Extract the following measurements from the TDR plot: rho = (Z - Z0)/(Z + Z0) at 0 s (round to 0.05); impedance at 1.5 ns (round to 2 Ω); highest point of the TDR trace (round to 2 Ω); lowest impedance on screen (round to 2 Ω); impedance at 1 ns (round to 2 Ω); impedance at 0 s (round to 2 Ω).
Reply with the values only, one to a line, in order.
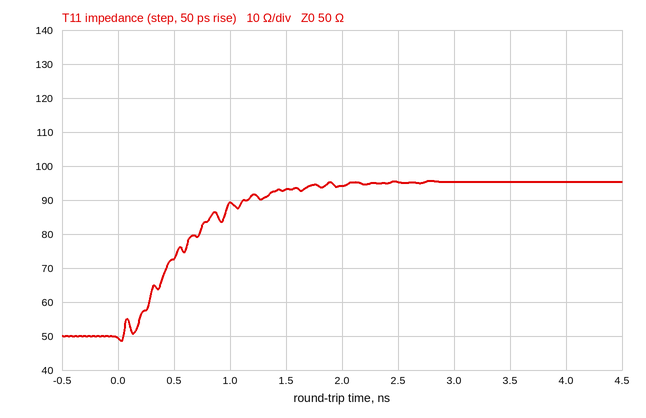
0.00
94 Ω
96 Ω
48 Ω
90 Ω
50 Ω
